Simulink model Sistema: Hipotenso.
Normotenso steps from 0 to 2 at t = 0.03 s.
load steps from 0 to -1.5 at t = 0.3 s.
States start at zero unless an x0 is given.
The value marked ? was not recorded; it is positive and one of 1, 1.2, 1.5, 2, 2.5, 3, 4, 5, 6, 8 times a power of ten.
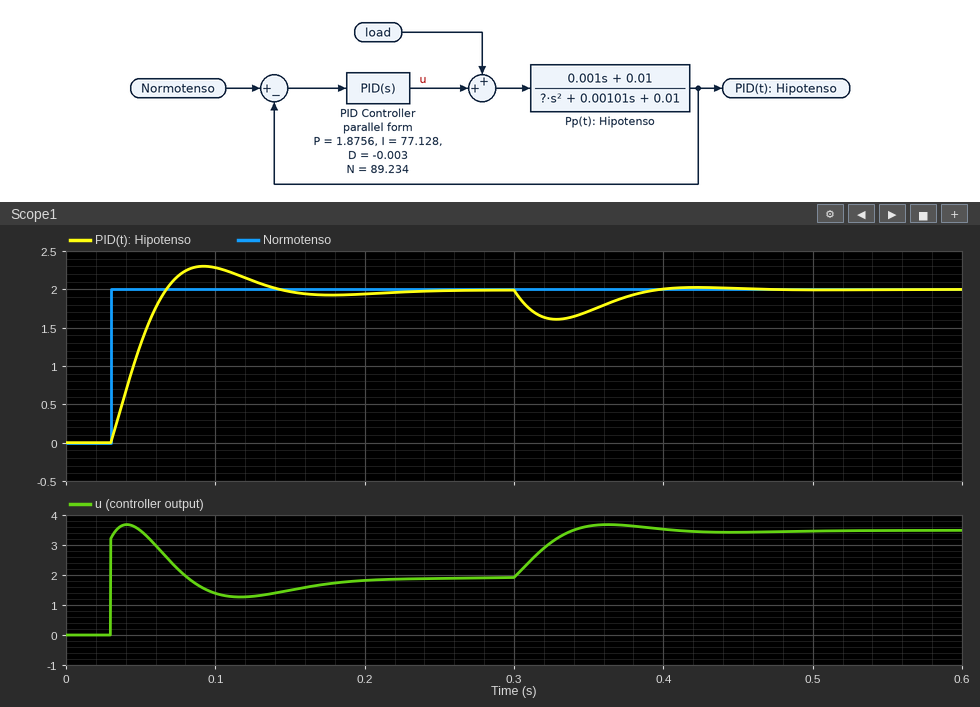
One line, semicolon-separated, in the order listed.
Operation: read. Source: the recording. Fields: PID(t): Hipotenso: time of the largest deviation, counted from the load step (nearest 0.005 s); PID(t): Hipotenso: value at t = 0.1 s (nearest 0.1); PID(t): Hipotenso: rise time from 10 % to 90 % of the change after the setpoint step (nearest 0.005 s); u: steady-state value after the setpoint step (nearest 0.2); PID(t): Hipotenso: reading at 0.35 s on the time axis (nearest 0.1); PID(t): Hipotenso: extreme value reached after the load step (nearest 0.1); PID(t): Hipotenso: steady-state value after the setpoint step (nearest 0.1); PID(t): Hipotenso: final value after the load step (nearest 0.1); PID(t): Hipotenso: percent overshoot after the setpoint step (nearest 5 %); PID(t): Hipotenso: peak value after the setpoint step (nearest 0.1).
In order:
0.030 s; 2.3; 0.030 s; 2.0; 1.7; 1.6; 2.0; 2.0; 15 %; 2.3
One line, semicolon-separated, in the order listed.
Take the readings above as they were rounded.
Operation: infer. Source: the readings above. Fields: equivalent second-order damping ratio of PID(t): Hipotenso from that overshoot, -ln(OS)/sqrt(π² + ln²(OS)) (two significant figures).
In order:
0.52
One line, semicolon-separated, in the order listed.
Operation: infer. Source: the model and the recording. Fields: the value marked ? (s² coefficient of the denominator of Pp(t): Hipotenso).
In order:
5e-05
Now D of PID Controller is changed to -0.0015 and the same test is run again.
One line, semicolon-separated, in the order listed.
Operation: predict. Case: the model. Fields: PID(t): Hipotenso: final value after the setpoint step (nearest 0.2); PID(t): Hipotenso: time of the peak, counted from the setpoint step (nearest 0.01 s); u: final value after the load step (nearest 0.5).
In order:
2.0; 0.06 s; 3.5
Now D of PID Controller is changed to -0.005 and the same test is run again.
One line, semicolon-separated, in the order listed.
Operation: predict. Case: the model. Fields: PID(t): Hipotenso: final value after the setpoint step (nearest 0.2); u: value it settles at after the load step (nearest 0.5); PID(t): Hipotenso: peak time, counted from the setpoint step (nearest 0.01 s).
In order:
2.0; 3.5; 0.06 s
